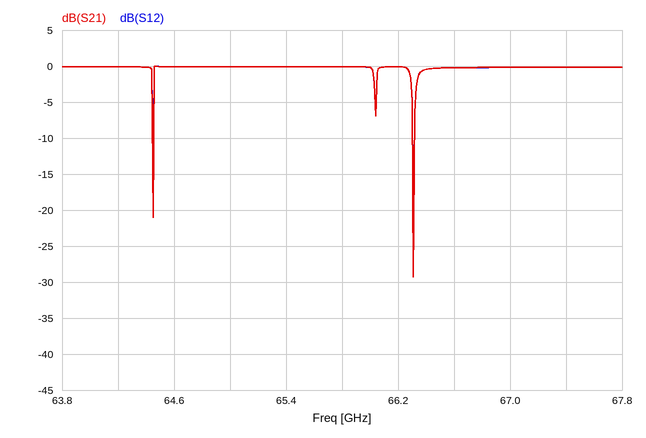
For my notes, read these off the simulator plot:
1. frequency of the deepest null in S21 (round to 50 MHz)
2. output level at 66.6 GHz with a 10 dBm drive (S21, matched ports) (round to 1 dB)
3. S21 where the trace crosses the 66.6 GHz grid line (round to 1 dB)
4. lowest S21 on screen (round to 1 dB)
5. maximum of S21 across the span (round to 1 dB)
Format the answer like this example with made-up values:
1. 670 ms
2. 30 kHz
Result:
1. 66.30 GHz
2. 10 dBm
3. 0 dB
4. -29 dB
5. 0 dB
